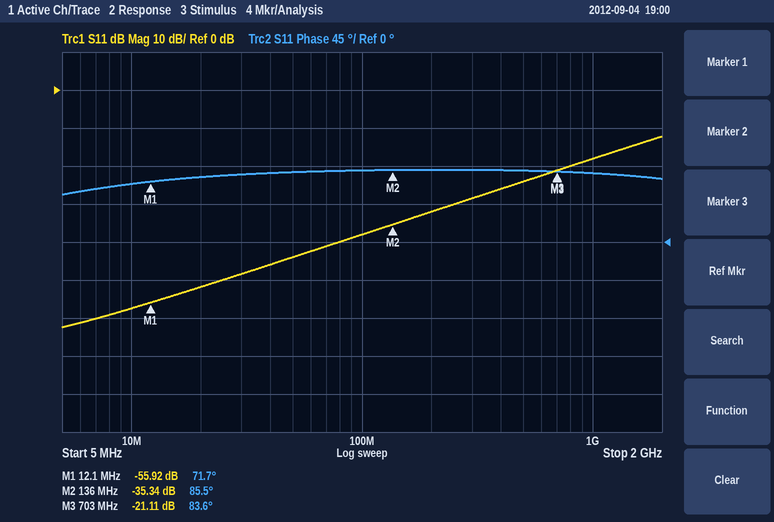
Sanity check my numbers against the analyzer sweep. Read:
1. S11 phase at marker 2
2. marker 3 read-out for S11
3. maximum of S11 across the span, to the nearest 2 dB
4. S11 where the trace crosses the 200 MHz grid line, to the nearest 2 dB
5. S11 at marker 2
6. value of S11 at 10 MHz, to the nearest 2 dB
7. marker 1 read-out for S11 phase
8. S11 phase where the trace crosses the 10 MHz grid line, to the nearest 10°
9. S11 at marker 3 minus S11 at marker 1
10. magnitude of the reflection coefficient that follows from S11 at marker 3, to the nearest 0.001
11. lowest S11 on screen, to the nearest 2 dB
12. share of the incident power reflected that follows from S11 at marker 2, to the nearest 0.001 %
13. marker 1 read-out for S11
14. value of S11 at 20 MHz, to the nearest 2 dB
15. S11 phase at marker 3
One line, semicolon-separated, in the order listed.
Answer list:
85.5°; -21.11 dB; -12 dB; -32 dB; -35.34 dB; -58 dB; 71.7°; 70°; 34.81 dB; 0.088; -62 dB; 0.029 %; -55.92 dB; -52 dB; 83.6°
